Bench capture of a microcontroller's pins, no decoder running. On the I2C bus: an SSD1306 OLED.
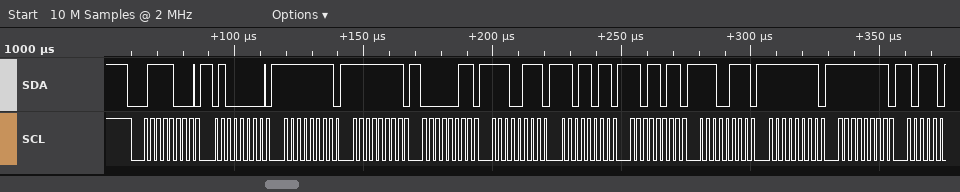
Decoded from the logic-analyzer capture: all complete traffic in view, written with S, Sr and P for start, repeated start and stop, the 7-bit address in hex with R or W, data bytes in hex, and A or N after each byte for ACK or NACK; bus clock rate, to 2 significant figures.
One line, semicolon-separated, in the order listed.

S 3CW A 40 A FF A FF A 03 A E7 A DB A DB A E7 A FF A FF A; 400 kHz
